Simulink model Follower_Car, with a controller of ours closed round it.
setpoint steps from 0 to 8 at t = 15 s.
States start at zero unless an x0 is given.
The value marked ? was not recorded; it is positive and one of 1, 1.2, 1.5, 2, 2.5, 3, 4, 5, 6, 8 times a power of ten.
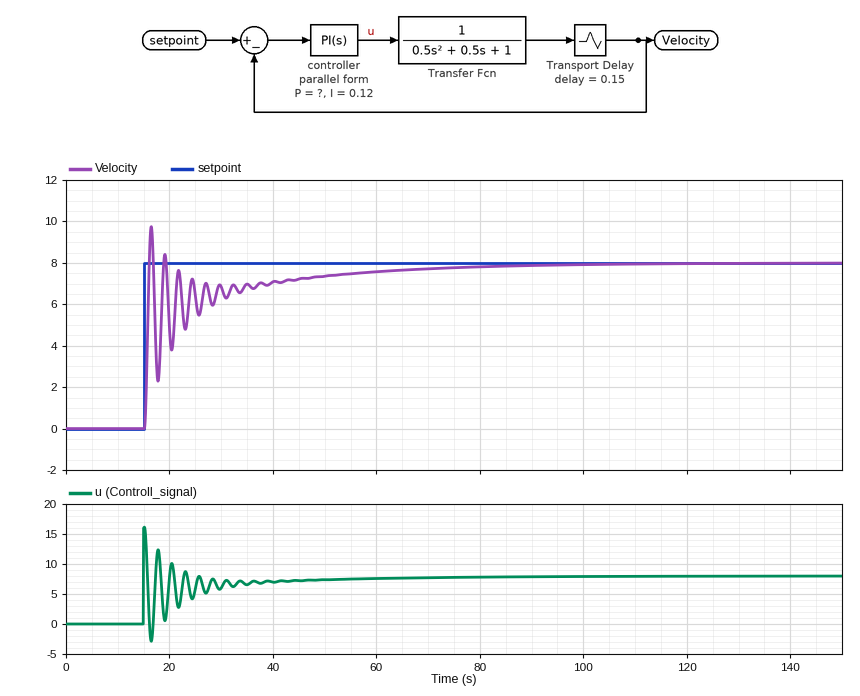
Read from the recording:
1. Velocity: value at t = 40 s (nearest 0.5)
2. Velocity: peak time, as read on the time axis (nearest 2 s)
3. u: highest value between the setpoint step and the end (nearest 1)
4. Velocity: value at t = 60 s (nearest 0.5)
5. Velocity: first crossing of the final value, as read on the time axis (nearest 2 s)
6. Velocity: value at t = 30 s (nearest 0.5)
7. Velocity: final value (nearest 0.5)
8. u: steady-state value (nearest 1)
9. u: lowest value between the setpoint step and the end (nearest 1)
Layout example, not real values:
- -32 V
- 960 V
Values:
- 7.0
- 16 s
- 16
- 7.5
- 16 s
- 7.0
- 8.0
- 8
- -3
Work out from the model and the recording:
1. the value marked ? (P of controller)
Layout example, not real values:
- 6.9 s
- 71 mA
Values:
- 2
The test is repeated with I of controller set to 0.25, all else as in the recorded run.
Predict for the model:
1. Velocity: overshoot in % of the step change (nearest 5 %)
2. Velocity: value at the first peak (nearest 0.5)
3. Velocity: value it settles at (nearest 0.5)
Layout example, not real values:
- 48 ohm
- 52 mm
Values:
- 25 %
- 10.0
- 8.0
